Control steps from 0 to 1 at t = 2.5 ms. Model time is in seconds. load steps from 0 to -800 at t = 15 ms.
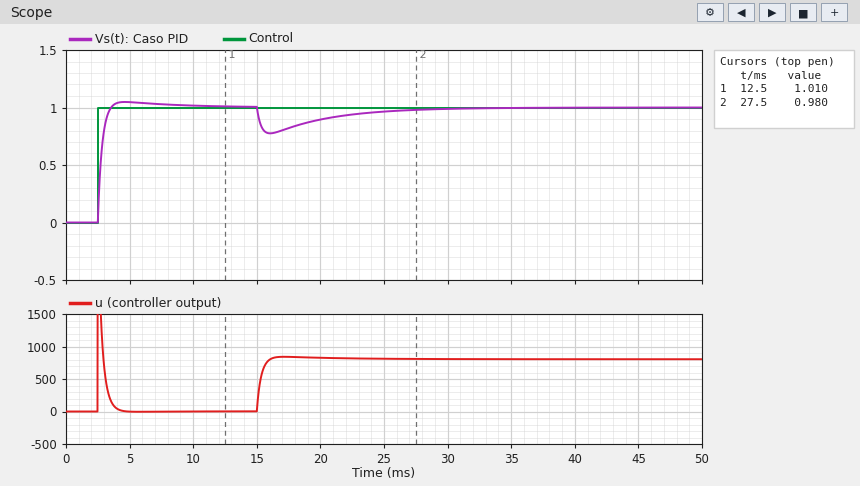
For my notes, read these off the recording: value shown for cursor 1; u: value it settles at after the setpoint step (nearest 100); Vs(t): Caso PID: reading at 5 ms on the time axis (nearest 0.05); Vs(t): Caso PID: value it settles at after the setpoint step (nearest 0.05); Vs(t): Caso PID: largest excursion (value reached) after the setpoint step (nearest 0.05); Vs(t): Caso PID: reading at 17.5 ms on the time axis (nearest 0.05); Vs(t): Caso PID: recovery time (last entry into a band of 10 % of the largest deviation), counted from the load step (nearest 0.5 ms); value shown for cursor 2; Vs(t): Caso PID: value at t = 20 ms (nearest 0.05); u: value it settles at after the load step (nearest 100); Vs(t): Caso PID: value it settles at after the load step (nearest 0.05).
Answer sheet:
1.010
0
1.05
1.00
1.05
0.80
12.0 ms
0.980
0.90
800
1.00
